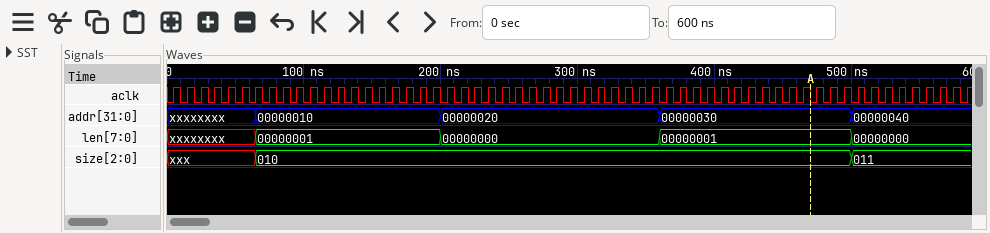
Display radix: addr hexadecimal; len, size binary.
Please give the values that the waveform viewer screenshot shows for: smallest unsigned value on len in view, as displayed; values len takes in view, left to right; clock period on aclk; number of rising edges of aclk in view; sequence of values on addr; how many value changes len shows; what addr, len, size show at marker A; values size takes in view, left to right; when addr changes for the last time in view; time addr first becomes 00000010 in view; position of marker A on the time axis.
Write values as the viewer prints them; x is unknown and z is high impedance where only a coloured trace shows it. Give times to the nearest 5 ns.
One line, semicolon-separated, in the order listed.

00000000; xxxxxxxx, 00000001, 00000000, 00000001, 00000000; 10 ns; 59; xxxxxxxx, 00000010, 00000020, 00000030, 00000040; 4; addr=00000030, len=00000001, size=010; xxx, 010, 011; 500 ns; 65 ns; 470 ns
